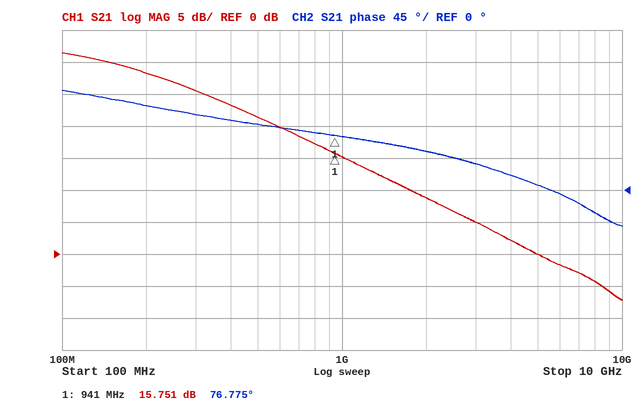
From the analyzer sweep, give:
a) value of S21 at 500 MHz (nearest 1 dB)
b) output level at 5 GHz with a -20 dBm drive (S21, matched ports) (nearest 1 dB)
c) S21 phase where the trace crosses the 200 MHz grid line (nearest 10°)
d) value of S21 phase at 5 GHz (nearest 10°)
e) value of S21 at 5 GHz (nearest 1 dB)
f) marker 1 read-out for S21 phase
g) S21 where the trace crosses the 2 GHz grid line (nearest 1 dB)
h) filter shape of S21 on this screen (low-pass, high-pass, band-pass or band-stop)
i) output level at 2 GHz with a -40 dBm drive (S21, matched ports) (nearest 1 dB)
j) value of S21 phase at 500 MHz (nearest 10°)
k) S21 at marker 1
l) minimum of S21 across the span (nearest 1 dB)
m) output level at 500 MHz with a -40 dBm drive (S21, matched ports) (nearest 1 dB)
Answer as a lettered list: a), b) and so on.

a) 21 dB
b) -20 dBm
c) 120°
d) 10°
e) 0 dB
f) 76.775°
g) 9 dB
h) low-pass
i) -31 dBm
j) 90°
k) 15.751 dB
l) -7 dB
m) -19 dBm
